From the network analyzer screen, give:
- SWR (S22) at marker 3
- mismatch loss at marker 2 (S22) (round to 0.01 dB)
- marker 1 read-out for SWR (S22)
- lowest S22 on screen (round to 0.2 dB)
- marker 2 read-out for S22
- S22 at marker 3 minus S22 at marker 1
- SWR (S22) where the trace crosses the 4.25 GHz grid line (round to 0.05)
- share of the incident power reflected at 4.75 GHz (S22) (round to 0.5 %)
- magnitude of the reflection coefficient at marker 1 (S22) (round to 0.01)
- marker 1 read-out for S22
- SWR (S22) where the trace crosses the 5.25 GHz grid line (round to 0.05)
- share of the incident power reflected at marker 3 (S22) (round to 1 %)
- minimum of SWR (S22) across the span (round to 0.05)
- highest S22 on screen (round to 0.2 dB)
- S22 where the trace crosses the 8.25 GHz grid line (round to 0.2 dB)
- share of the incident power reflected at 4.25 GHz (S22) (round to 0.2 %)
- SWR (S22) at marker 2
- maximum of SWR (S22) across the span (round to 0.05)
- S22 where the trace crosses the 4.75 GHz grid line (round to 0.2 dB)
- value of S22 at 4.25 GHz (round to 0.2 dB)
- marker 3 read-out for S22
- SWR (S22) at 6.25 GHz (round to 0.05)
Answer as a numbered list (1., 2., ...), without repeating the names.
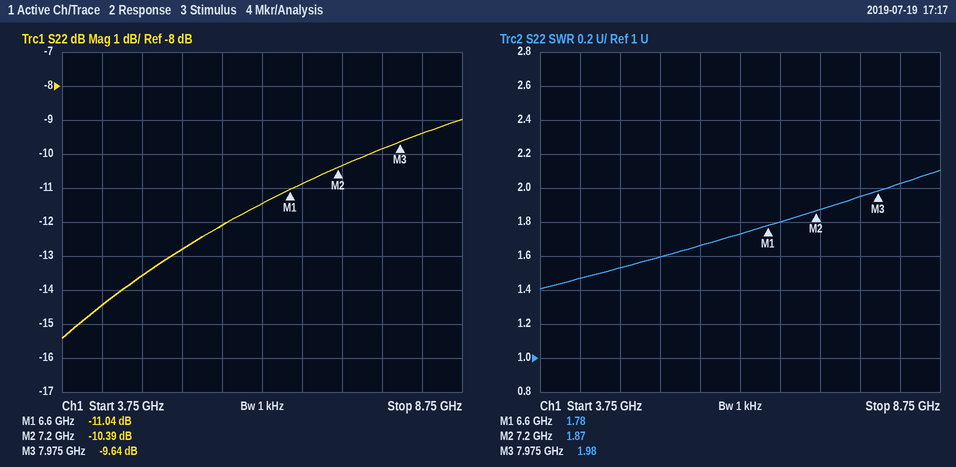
1. 1.98
2. 0.42 dB
3. 1.78
4. -15.4 dB
5. -10.39 dB
6. 1.40 dB
7. 1.45
8. 4.5 %
9. 0.28
10. -11.04 dB
11. 1.60
12. 11 %
13. 1.40
14. -9.0 dB
15. -9.4 dB
16. 3.6 %
17. 1.87
18. 2.10
19. -13.6 dB
20. -14.4 dB
21. -9.64 dB
22. 1.75
